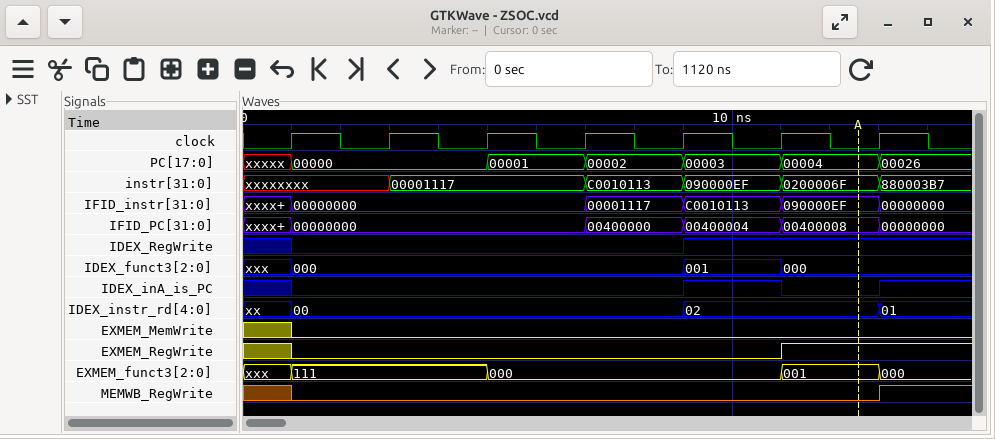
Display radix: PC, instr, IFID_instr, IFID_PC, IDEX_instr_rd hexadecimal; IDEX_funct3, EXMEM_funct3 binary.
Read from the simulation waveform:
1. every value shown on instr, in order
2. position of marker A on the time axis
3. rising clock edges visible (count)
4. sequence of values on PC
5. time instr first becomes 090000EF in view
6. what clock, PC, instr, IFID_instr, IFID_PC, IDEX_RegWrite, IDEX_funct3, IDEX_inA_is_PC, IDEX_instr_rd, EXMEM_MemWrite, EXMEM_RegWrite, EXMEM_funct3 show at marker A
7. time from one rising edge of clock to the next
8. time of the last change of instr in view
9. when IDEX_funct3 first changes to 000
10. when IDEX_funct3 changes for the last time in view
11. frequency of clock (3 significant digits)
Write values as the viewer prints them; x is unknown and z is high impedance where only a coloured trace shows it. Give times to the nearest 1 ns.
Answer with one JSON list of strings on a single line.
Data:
["xxxxxxxx, 00001117, C0010113, 090000EF, 0200006F, 880003B7", "13 ns", "7", "xxxxx, 00000, 00001, 00002, 00003, 00004, 00026", "9 ns", "clock=0, PC=00004, instr=0200006F, IFID_instr=090000EF, IFID_PC=00400008, IDEX_RegWrite=1, IDEX_funct3=000, IDEX_inA_is_PC=0, IDEX_instr_rd=02, EXMEM_MemWrite=0, EXMEM_RegWrite=1, EXMEM_funct3=001", "2 ns", "13 ns", "1 ns", "11 ns", "500 MHz"]
